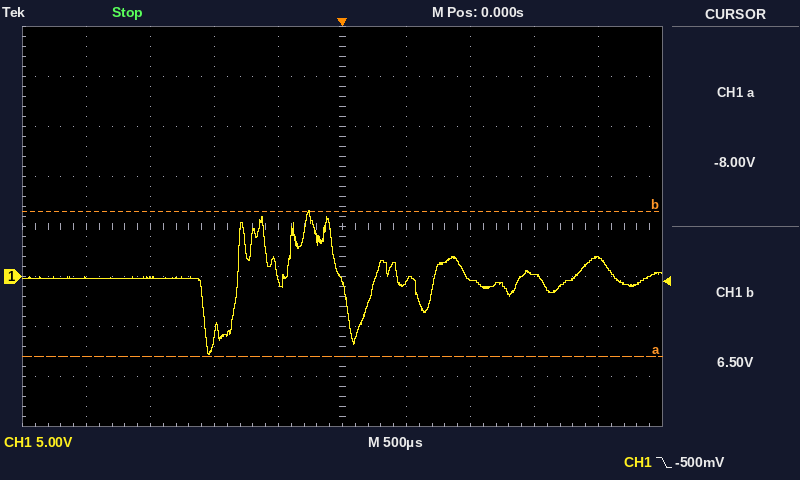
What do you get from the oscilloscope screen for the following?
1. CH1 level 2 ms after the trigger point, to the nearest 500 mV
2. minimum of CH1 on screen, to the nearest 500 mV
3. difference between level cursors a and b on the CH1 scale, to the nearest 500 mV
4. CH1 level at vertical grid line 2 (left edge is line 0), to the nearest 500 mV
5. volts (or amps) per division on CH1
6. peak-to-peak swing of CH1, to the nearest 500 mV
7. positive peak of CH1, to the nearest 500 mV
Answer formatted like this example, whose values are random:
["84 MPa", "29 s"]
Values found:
["2.0 V", "-8.0 V", "14.5 V", "0.0 V", "5 V", "14.5 V", "6.5 V"]
